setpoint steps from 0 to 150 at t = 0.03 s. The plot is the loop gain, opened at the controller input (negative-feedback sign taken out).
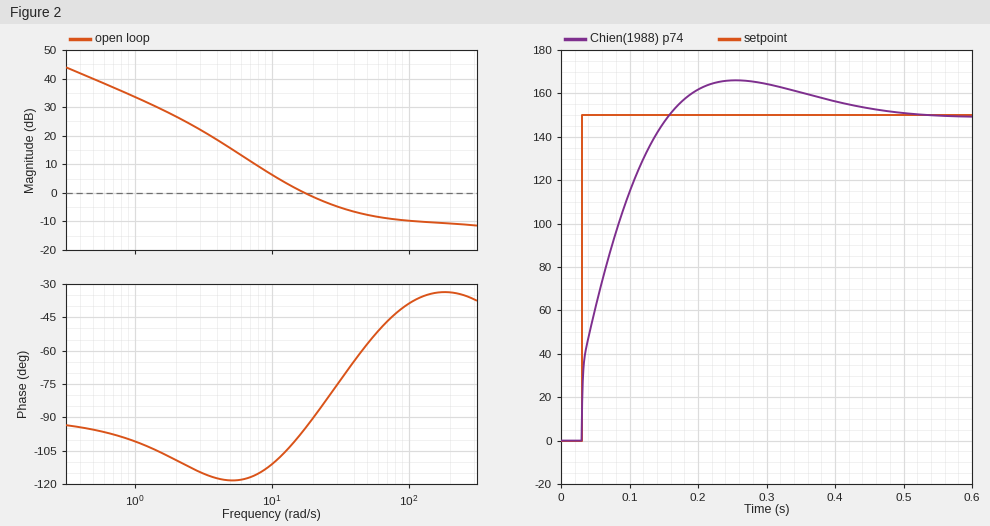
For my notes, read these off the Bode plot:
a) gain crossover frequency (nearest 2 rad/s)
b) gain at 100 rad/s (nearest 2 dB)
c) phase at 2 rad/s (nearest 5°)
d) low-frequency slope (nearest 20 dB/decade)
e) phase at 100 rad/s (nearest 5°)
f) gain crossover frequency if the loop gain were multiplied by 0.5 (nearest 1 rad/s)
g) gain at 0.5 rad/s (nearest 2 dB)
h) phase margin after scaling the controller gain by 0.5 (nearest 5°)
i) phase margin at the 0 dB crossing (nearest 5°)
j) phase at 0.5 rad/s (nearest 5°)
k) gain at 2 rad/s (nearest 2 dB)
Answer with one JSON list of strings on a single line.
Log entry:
["18 rad/s", "-10 dB", "-110°", "-20 dB/decade", "-40°", "10 rad/s", "40 dB", "70°", "85°", "-95°", "26 dB"]
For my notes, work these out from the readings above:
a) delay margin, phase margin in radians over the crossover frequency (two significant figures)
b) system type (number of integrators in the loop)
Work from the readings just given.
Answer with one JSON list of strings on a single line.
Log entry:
["0.082 s", "1"]
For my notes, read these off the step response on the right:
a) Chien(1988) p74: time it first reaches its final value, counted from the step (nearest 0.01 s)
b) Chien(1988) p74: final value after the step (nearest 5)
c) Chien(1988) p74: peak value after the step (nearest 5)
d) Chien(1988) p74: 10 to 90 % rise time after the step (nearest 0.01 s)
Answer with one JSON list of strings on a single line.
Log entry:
["0.13 s", "150", "165", "0.10 s"]
